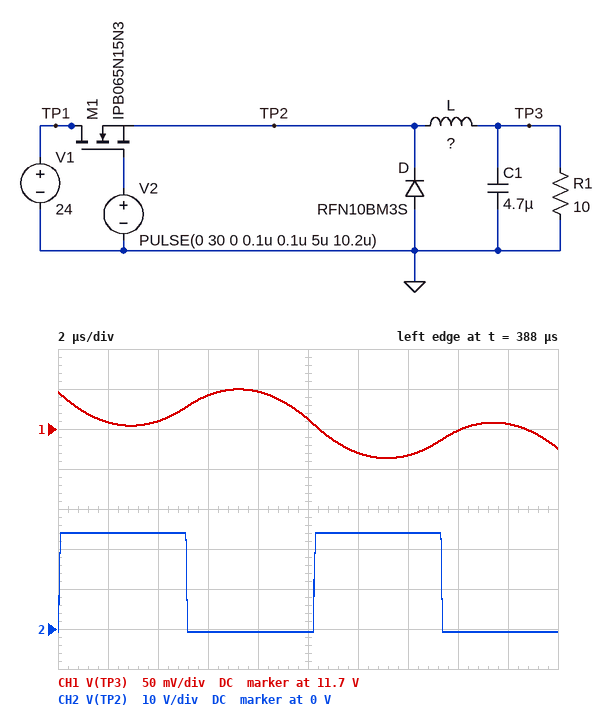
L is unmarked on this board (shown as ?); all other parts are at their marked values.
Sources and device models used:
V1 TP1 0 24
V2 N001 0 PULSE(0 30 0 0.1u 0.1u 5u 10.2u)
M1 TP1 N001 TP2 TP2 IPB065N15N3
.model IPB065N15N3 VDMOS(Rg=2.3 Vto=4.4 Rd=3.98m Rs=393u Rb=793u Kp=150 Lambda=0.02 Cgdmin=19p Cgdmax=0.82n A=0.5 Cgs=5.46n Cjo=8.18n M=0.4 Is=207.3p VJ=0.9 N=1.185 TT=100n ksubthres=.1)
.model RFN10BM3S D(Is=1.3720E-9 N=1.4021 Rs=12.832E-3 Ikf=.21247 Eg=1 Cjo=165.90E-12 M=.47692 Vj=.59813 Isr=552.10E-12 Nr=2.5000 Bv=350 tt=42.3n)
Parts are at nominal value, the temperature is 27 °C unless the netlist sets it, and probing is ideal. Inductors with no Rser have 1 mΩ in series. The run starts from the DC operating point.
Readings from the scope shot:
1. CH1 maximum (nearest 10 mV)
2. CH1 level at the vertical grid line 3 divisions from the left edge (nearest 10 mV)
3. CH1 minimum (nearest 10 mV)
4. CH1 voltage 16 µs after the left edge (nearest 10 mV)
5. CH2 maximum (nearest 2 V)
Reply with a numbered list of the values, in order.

1. 11.75 V
2. 11.74 V
3. 11.66 V
4. 11.70 V
5. 24 V
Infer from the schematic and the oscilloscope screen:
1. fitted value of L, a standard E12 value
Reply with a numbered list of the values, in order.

1. 270 µH
